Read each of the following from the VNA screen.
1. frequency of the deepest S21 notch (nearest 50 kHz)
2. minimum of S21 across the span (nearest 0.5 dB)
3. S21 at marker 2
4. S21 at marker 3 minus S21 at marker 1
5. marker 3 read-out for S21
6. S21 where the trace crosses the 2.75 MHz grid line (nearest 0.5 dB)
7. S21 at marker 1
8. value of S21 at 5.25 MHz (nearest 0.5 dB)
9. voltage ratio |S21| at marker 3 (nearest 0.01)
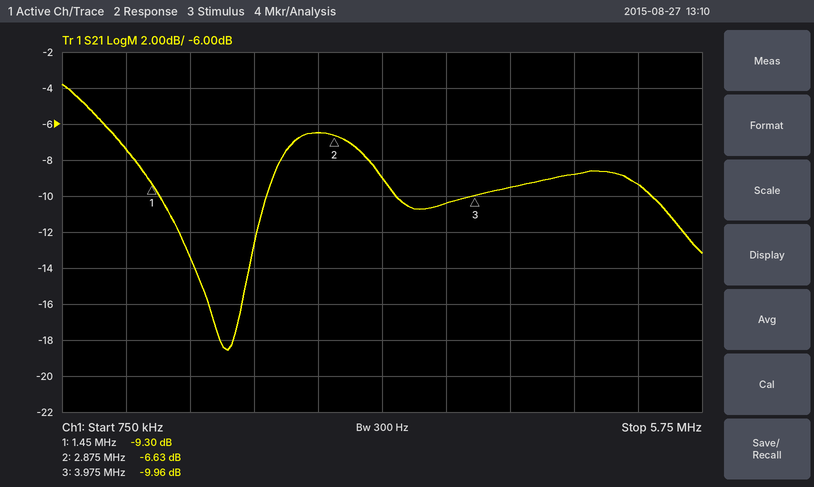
2.05 MHz
-18.5 dB
-6.63 dB
-0.66 dB
-9.96 dB
-6.5 dB
-9.30 dB
-9.5 dB
0.32
